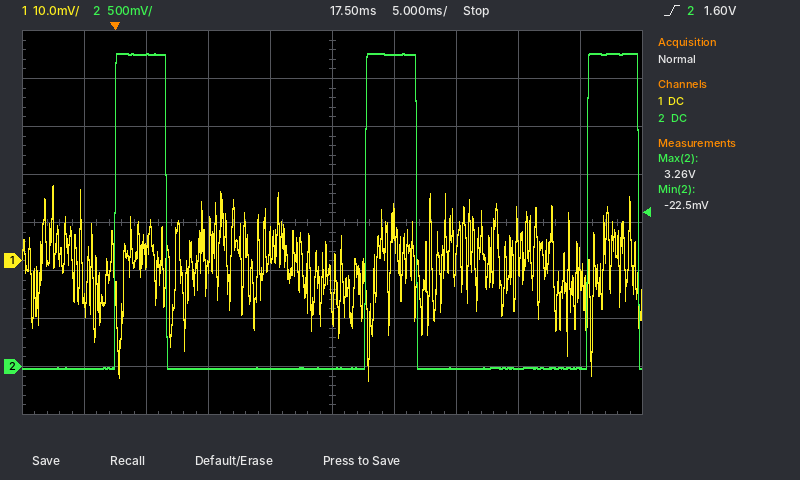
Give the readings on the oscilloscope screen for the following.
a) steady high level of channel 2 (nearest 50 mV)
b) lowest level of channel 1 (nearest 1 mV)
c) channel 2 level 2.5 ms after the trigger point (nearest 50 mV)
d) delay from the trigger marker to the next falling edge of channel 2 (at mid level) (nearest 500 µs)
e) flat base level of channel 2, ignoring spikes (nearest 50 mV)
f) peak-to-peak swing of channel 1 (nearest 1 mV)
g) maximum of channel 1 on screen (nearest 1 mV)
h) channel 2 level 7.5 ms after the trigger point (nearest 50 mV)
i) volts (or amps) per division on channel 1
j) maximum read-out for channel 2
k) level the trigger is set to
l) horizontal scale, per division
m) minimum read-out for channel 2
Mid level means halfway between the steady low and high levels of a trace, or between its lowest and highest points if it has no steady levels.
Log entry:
3.25 V
-25 mV
3.25 V
4.0 ms
0 mV
41 mV
16 mV
0 mV
10 mV
3.26 V
1.60 V
5 ms
-22.5 mV
